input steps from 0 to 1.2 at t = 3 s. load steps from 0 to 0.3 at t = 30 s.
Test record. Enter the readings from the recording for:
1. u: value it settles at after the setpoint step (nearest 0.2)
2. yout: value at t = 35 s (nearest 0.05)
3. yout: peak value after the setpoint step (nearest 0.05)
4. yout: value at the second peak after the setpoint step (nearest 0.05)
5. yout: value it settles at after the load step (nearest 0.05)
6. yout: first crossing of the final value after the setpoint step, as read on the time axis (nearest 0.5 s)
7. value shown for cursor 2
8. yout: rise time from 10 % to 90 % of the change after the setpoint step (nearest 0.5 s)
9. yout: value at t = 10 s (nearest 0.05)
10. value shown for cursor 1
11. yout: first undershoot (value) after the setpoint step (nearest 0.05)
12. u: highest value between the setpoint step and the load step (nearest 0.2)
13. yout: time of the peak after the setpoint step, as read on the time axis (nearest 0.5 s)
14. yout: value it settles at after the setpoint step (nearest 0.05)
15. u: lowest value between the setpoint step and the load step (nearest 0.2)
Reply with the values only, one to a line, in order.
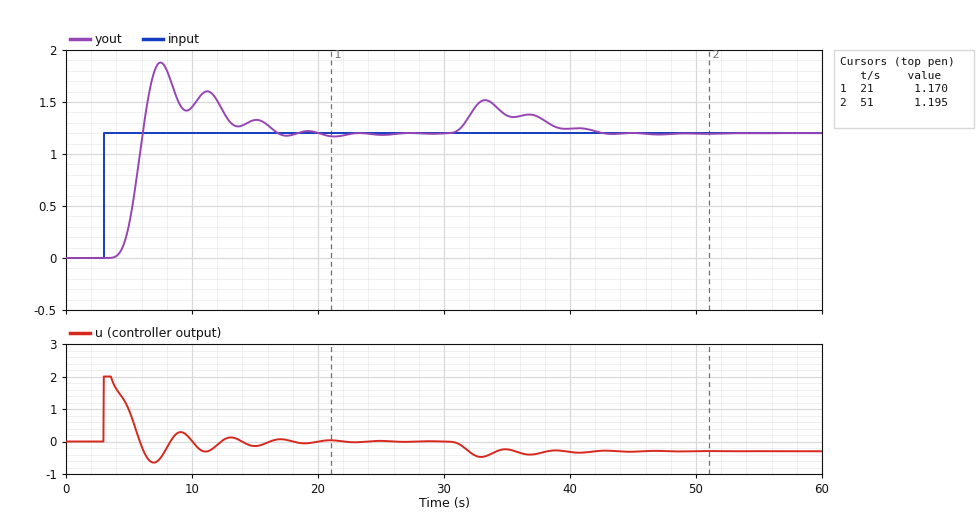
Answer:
0.0
1.35
1.90
1.60
1.20
6.0 s
1.195
1.5 s
1.45
1.170
1.40
2.0
7.5 s
1.20
-0.6
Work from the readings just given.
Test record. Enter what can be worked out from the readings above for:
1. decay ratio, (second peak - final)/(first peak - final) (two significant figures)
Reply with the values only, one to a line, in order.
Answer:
0.57
